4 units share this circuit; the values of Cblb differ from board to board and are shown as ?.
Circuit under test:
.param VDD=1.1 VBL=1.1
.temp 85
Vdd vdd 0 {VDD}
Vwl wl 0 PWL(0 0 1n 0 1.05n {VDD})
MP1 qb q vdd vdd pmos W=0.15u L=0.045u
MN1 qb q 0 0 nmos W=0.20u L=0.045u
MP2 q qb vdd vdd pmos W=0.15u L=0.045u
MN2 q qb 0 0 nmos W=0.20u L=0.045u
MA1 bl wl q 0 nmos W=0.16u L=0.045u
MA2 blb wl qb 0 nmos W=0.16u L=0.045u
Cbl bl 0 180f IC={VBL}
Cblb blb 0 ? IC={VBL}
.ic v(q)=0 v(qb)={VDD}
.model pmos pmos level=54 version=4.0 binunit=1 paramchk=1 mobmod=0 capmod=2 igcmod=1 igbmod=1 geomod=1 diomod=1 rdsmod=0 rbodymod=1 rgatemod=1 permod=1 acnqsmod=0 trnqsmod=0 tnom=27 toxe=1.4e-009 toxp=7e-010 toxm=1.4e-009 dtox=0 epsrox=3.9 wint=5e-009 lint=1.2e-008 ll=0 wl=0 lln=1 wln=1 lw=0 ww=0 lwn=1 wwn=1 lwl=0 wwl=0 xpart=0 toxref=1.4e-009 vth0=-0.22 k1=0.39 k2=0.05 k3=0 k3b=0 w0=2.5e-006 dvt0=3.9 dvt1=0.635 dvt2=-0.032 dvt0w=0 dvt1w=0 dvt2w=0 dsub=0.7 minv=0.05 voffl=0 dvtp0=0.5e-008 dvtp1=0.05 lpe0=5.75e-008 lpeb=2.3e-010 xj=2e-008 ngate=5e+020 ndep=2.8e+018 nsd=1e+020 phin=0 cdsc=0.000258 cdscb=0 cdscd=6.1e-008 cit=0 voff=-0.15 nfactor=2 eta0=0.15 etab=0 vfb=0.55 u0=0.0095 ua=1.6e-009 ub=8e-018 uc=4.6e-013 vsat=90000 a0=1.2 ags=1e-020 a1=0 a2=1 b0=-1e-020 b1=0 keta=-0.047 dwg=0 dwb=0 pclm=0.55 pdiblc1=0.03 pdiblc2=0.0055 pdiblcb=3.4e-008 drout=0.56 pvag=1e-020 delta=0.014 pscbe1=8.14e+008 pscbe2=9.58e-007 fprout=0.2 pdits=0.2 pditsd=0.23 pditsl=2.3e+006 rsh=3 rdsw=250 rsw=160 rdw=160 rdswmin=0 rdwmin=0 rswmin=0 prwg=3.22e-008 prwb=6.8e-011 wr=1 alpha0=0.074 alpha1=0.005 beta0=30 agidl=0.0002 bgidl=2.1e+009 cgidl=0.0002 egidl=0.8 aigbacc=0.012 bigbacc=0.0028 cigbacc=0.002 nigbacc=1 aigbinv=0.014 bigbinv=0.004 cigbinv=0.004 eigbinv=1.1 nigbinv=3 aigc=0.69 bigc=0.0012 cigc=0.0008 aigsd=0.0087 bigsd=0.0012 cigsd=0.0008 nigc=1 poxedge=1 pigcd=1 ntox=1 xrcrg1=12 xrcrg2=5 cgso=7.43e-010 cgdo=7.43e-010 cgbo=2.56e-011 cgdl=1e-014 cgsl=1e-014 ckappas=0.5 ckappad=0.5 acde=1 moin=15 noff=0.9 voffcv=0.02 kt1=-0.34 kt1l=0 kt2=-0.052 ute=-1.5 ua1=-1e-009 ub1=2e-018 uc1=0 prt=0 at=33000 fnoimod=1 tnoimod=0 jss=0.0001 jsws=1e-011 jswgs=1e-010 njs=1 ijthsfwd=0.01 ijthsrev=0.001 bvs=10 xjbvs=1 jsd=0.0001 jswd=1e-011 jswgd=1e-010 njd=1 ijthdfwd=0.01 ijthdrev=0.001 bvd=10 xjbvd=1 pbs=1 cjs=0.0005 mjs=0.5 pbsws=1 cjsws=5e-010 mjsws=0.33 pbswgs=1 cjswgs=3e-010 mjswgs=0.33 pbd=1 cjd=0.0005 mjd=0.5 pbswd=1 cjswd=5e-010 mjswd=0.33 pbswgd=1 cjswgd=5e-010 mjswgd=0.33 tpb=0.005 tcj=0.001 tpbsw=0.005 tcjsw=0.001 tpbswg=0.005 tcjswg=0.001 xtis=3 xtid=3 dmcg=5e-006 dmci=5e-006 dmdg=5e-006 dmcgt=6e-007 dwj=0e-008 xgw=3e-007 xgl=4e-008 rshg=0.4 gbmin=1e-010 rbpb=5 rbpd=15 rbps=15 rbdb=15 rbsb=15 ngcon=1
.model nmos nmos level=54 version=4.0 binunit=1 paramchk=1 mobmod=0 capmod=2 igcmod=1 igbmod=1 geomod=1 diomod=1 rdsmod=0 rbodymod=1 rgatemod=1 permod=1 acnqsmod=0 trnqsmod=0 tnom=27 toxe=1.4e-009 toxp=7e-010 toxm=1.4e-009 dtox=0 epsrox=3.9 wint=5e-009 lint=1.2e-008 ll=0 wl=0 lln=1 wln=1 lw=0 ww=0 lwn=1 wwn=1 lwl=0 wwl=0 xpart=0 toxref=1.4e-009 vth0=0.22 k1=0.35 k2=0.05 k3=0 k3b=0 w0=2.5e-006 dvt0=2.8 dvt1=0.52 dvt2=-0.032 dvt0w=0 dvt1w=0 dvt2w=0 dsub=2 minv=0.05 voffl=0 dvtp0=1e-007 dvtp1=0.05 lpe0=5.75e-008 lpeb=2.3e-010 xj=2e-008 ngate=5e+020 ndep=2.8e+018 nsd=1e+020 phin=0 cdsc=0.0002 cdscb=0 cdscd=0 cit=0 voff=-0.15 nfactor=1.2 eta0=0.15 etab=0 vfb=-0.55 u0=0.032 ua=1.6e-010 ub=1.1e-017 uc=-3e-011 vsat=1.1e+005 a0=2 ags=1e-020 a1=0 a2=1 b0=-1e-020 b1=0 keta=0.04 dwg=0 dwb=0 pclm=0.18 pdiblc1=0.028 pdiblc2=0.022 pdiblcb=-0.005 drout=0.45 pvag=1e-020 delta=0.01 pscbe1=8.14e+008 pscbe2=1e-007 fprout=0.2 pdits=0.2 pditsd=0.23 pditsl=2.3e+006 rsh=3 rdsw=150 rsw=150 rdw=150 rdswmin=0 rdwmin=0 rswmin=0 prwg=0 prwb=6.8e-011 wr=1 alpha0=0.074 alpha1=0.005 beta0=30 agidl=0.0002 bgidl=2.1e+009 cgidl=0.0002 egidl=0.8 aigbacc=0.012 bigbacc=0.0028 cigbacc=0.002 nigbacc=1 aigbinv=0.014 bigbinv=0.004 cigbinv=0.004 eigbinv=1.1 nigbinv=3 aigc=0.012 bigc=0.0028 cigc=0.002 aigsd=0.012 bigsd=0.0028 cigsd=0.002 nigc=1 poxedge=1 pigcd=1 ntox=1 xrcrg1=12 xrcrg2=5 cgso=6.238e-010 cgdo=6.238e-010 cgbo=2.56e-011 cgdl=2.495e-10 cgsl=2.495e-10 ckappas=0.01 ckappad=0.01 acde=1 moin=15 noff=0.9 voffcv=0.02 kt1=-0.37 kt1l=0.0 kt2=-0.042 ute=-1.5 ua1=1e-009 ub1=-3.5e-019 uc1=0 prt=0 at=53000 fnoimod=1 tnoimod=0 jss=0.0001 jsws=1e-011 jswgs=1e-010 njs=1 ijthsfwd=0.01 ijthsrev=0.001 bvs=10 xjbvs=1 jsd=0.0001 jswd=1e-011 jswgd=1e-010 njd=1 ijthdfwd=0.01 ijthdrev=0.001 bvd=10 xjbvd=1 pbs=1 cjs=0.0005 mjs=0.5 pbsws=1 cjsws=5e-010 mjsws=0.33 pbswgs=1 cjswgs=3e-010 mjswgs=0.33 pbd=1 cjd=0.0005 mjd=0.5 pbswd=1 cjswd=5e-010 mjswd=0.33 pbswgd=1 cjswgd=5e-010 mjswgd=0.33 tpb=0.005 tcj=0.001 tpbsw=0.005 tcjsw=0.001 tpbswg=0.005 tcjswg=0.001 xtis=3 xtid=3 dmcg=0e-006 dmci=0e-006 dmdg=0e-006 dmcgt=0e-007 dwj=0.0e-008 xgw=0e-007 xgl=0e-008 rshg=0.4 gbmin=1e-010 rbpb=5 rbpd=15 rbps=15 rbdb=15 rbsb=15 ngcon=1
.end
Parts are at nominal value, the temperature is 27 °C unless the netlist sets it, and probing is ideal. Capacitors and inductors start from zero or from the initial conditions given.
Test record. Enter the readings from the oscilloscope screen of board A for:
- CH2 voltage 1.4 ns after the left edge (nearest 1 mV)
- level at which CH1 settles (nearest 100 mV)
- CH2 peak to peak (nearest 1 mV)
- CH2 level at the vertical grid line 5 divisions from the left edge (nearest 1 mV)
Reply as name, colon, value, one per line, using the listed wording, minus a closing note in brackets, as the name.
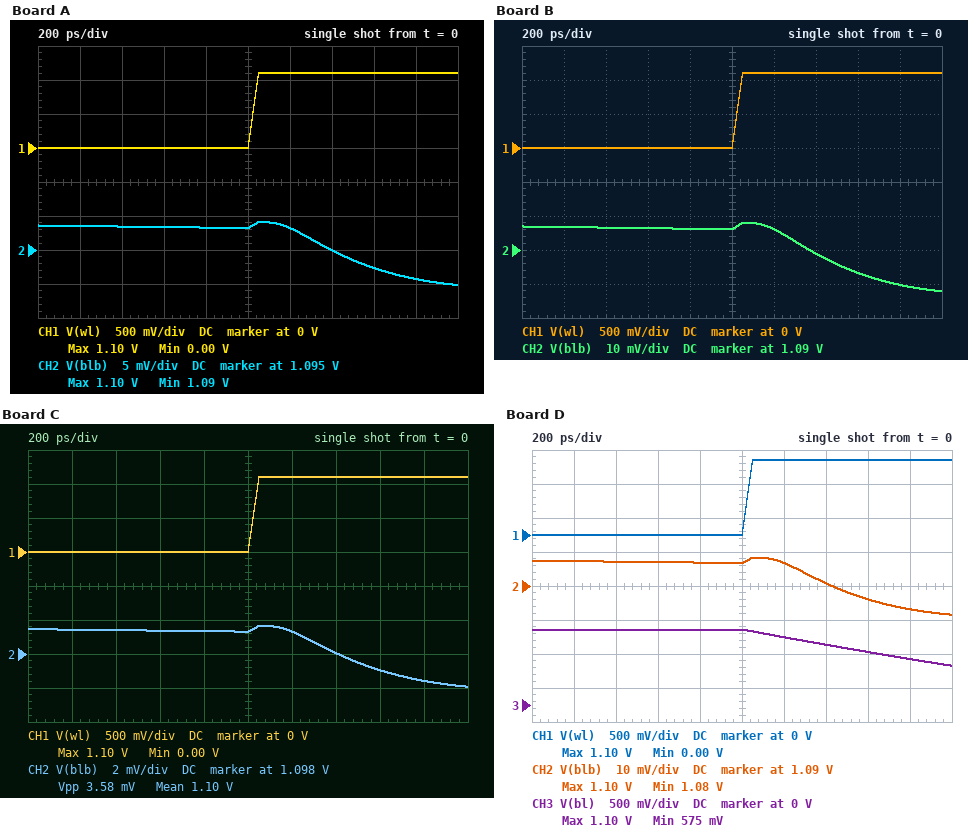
CH2 voltage 1.4 ns after the left edge: 1.095 V
level at which CH1 settles: 1.1 V
CH2 peak to peak: 9 mV
CH2 level at the vertical grid line 5 divisions from the left edge: 1.098 V
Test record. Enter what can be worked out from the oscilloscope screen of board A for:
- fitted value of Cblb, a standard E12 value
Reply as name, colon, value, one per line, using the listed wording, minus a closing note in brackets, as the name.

fitted value of Cblb, a standard E12 value: 150 fF
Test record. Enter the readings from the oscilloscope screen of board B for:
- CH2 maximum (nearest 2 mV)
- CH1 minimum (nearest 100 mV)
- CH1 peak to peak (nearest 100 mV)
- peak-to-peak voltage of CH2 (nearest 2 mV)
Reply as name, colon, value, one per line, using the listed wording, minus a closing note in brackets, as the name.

CH2 maximum: 1.098 V
CH1 minimum: 0 V
CH1 peak to peak: 1.1 V
peak-to-peak voltage of CH2: 20 mV
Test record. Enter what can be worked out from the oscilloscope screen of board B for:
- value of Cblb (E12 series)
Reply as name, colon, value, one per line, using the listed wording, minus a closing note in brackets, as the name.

value of Cblb: 68 fF
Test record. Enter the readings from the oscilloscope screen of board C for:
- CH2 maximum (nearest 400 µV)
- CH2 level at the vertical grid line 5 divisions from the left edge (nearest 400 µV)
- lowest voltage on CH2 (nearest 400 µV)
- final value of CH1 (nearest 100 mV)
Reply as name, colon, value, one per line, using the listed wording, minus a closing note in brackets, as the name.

CH2 maximum: 1.0996 V
CH2 level at the vertical grid line 5 divisions from the left edge: 1.0992 V
lowest voltage on CH2: 1.0960 V
final value of CH1: 1.1 V
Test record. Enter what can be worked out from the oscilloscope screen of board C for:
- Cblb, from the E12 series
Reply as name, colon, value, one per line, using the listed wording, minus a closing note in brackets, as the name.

Cblb, from the E12 series: 390 fF
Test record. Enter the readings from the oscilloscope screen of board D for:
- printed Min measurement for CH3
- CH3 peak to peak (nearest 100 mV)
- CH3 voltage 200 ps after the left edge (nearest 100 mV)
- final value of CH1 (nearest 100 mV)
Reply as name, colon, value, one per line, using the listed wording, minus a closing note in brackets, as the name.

printed Min measurement for CH3: 575 mV
CH3 peak to peak: 500 mV
CH3 voltage 200 ps after the left edge: 1.1 V
final value of CH1: 1.1 V
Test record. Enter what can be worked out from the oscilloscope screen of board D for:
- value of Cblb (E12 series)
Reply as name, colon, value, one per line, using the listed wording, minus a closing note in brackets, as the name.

value of Cblb: 82 fF
